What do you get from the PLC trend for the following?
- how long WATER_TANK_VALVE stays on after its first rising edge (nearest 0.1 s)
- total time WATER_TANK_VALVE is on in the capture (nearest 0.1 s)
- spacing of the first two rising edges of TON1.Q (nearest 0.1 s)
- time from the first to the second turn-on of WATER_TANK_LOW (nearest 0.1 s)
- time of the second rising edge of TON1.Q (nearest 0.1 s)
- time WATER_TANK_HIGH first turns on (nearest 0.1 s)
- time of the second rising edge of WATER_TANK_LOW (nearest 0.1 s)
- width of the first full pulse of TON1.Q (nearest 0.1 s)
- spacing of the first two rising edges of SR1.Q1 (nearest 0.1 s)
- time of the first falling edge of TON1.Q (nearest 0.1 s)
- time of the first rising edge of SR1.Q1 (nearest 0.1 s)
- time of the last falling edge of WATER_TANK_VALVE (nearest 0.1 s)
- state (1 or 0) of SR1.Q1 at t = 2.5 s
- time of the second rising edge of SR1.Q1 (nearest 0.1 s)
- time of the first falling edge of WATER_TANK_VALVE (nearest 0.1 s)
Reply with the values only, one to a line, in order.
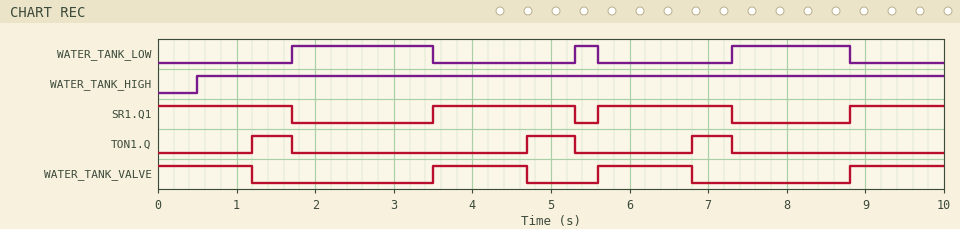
1.2 s
4.8 s
3.5 s
3.6 s
4.7 s
0.5 s
5.3 s
0.5 s
2.1 s
1.7 s
3.5 s
6.8 s
0
5.6 s
1.2 s
